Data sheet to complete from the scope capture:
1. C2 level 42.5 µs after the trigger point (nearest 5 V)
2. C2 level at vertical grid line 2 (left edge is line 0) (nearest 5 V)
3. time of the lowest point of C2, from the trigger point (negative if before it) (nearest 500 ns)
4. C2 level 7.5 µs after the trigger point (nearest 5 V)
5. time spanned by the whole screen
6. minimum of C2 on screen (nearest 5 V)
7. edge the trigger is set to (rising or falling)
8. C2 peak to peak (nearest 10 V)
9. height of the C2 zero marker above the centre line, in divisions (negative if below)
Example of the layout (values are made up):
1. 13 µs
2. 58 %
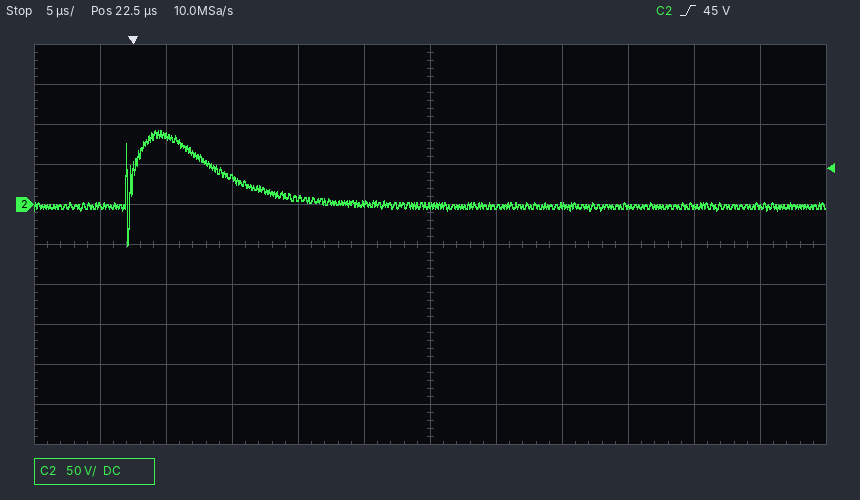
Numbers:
1. 0 V
2. 85 V
3. -500 ns
4. 35 V
5. 60 µs
6. -50 V
7. rising
8. 140 V
9. +1.0 div
